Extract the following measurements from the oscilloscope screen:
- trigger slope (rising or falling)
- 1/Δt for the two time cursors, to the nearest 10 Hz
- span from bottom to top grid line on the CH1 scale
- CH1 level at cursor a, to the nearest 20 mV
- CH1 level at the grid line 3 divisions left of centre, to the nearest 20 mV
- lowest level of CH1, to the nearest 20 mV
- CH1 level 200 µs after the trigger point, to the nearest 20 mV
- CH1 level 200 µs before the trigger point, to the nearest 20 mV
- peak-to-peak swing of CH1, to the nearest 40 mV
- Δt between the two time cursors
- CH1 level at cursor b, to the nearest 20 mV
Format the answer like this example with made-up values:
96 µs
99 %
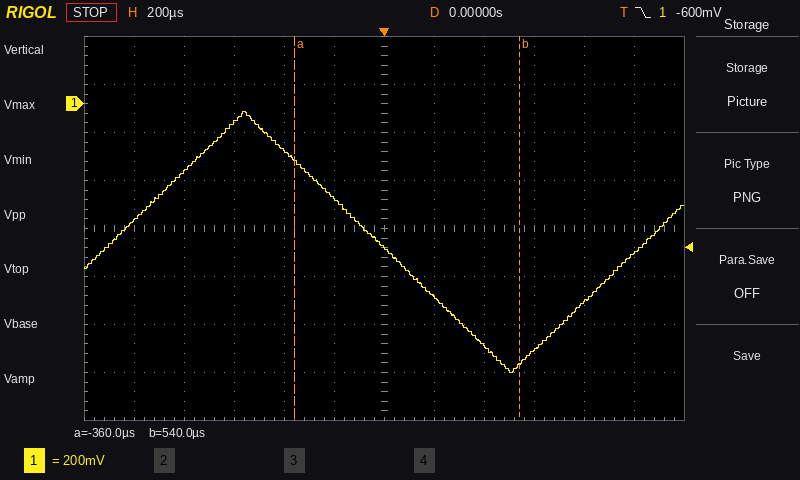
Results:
falling
1.11 kHz
1.6 V
-240 mV
-80 mV
-1.12 V
-800 mV
-400 mV
1.08 V
900 µs
-1.08 V
